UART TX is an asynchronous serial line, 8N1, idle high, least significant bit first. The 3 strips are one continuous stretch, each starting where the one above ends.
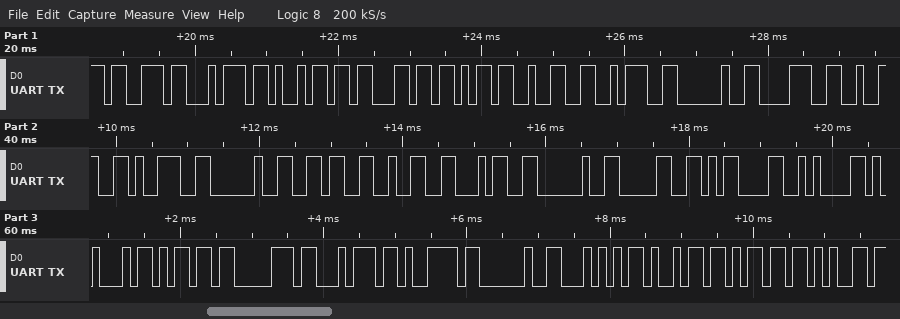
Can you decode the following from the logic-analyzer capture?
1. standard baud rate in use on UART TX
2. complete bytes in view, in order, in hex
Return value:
9600 baud
73 74 69 63 6B 32 3A 20 38 32 39 20 36 32 34 20 30 0D 0A 45 6D 70 74 79 20 54 69 6D 65
